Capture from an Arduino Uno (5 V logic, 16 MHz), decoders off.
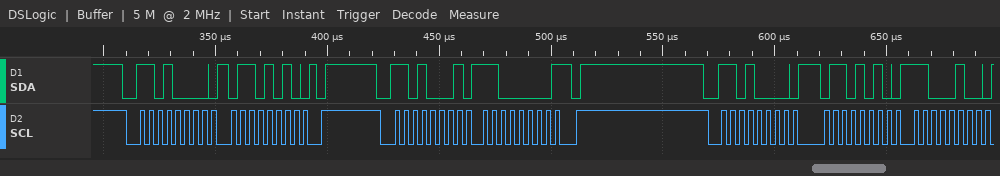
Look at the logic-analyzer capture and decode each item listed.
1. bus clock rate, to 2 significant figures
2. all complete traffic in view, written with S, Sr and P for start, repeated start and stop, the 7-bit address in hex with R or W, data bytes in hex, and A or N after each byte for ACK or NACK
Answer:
250 kHz
S 68W A 6A A P S 68R A C0 N P S 68W A 6A A C4 A
